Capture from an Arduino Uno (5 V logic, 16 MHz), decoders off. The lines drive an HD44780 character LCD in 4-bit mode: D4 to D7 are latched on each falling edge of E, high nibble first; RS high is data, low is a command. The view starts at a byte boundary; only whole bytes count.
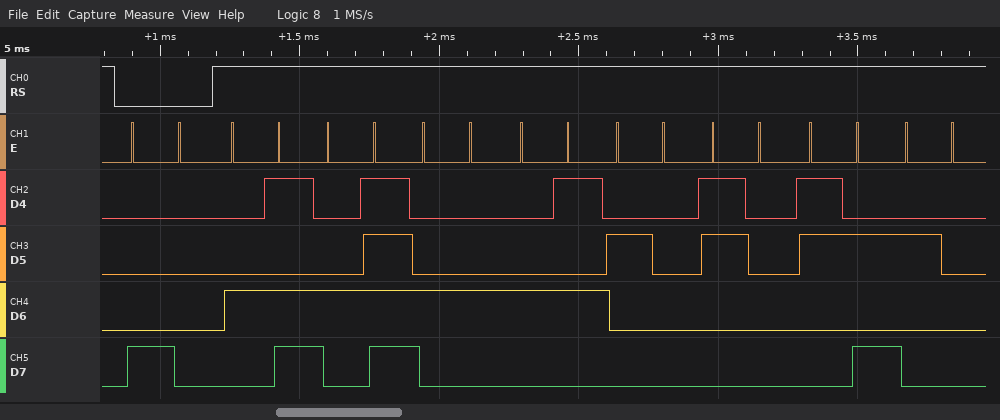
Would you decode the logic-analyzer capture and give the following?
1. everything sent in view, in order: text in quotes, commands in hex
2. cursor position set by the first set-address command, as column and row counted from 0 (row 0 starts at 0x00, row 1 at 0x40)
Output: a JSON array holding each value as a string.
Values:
["0x80 \"MODE 0: \"", "column 0, row 0"]
